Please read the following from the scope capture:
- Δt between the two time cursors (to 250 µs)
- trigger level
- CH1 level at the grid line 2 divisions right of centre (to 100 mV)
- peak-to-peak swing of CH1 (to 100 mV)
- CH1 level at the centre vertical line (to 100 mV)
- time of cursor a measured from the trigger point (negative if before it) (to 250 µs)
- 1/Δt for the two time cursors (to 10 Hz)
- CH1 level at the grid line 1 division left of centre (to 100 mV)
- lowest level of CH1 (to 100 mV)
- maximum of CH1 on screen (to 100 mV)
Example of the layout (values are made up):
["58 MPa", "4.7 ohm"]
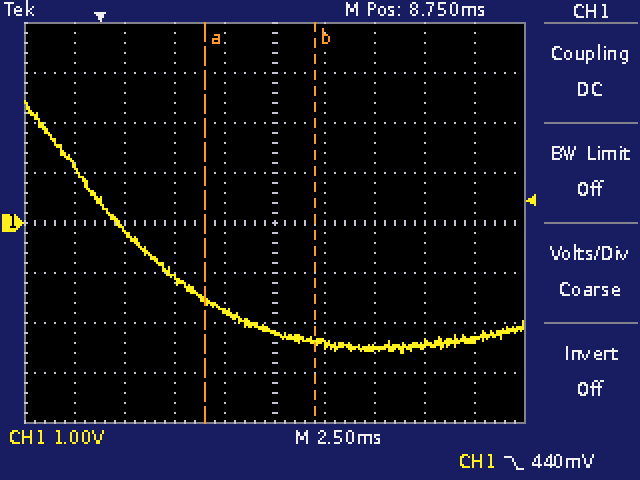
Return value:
["5.50 ms", "440 mV", "-2.5 V", "5.0 V", "-2.2 V", "+5.25 ms", "180 Hz", "-1.8 V", "-2.6 V", "2.4 V"]
